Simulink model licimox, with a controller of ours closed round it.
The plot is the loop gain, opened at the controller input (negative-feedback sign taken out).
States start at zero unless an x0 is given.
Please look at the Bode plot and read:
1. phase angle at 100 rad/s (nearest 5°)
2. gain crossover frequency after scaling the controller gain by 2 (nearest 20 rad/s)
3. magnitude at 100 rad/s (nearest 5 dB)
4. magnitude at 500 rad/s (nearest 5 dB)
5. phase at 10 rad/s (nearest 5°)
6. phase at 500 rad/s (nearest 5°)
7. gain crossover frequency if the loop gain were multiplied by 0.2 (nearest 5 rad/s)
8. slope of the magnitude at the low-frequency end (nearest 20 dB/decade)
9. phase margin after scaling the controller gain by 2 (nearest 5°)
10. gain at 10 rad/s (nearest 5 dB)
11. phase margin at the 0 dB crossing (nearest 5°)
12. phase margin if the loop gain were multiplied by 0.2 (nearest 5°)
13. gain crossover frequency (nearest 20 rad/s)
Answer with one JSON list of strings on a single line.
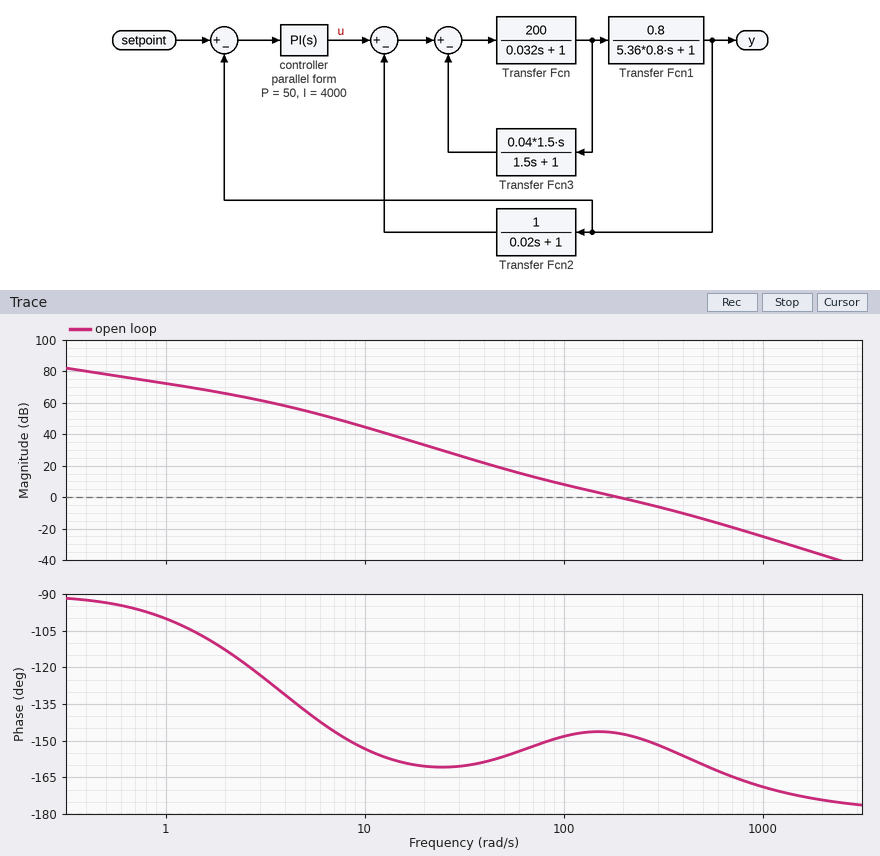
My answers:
["-150°", "300 rad/s", "10 dB", "-15 dB", "-155°", "-160°", "65 rad/s", "-20 dB/decade", "30°", "45 dB", "35°", "25°", "180 rad/s"]
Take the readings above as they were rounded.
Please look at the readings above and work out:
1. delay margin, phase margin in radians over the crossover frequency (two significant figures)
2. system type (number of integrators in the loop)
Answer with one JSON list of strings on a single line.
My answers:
["0.0034 s", "1"]
